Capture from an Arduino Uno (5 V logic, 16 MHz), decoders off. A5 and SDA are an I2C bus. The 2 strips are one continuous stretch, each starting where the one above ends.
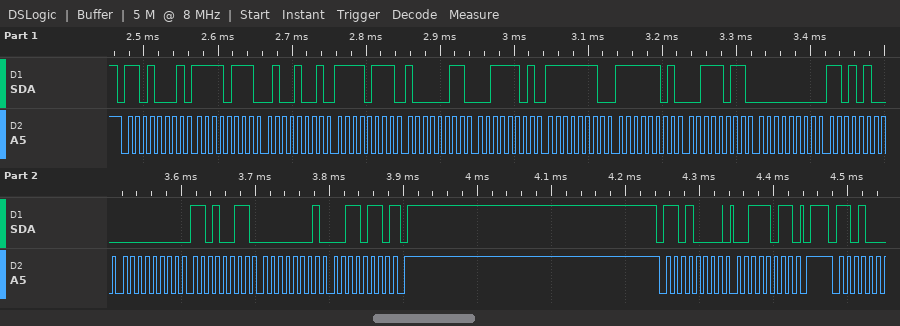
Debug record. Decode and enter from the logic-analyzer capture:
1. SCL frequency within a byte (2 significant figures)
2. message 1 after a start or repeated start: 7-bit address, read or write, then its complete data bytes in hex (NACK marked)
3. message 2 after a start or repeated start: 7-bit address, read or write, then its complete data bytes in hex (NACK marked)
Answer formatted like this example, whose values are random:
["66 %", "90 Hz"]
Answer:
["100 kHz", "0x68 read: F7 49 F7 83 3D FE FD 3B 00 D4 00 D3 01 36 NACK", "0x68 write: 3B"]
